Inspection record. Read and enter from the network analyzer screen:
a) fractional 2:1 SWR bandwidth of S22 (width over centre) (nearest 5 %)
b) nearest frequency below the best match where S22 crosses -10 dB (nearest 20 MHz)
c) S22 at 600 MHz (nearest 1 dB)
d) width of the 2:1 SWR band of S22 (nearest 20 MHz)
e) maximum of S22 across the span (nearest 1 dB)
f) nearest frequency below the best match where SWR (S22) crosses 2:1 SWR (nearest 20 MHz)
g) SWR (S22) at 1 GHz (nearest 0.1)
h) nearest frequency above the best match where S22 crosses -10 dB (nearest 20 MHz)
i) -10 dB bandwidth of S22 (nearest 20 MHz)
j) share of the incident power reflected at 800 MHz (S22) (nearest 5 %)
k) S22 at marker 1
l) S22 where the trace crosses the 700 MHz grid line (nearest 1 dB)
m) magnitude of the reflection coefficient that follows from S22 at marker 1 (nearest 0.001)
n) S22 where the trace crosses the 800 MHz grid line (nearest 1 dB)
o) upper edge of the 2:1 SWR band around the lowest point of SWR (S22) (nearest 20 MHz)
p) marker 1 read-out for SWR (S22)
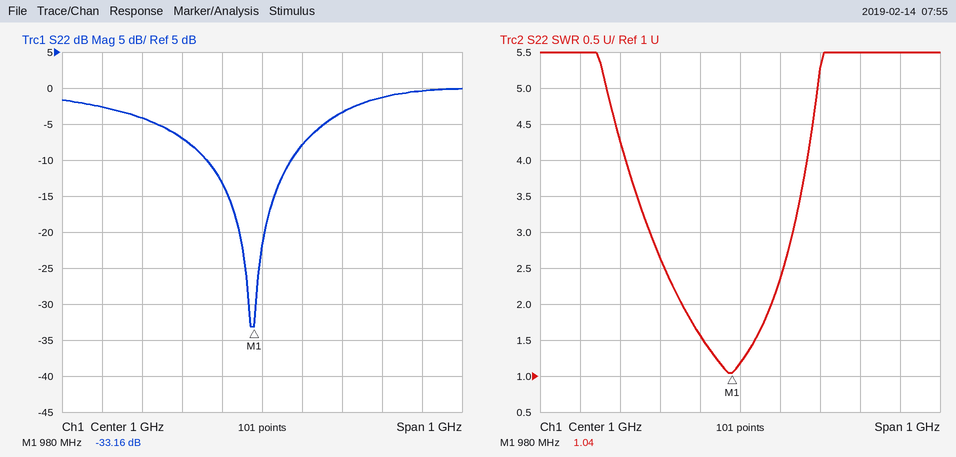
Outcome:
25 %
860 MHz
-3 dB
220 MHz
0 dB
860 MHz
1.2
1.08 GHz
220 MHz
20 %
-33.16 dB
-4 dB
0.022
-7 dB
1.08 GHz
1.04
